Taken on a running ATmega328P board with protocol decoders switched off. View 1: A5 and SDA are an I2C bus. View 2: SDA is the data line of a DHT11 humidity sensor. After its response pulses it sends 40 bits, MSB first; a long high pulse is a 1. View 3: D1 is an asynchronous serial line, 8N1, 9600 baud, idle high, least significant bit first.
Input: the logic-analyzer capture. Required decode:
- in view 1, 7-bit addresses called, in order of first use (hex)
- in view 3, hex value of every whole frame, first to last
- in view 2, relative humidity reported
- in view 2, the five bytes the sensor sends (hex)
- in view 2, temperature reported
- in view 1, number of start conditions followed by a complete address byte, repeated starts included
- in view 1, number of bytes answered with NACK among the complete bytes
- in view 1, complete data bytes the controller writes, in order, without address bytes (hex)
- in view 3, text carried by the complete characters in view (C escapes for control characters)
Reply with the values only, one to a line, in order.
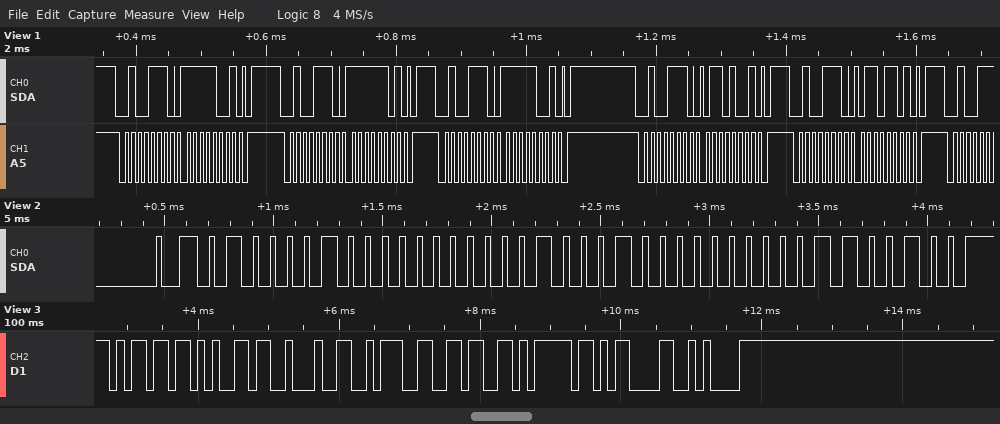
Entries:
0x27
6D 65 22 3A 36 7D 0D 0A
66 %
42 00 22 00 64
34.0 °C
5
0
F9 FD F9 69 6D
"me\":6}\r\n"
